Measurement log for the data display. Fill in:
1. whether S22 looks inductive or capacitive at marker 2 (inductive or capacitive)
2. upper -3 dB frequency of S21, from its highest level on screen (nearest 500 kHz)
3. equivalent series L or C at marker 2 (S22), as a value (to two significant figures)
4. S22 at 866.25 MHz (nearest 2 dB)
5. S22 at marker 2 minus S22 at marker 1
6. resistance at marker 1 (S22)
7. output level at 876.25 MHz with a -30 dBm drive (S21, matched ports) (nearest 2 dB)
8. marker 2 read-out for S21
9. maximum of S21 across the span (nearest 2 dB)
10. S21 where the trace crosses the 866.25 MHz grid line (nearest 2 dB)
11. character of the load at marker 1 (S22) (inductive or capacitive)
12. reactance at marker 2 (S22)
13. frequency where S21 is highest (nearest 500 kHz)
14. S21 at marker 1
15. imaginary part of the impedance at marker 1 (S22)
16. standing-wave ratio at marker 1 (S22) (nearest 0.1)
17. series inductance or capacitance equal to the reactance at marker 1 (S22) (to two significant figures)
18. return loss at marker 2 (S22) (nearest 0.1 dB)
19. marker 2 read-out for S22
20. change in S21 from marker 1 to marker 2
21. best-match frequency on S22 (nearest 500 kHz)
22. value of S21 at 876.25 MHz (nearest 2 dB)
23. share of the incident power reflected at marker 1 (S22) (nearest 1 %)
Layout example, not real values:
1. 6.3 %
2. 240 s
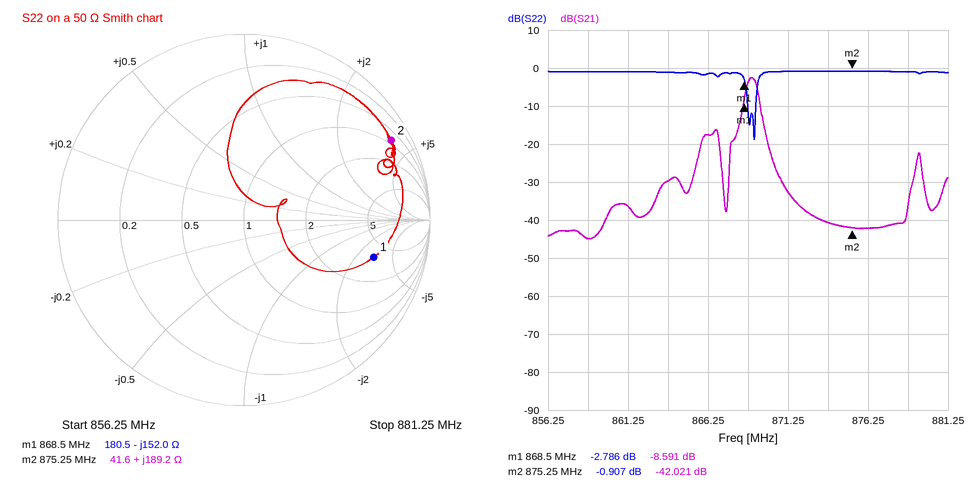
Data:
1. inductive
2. 869.5 MHz
3. 34 nH
4. -2 dB
5. 1.879 dB
6. 180.5 Ω
7. -72 dBm
8. -42.021 dB
9. -2 dB
10. -18 dB
11. capacitive
12. +189.2 Ω
13. 869.0 MHz
14. -8.591 dB
15. -152.0 Ω
16. 6.3
17. 1.2 pF
18. 0.9 dB
19. -0.907 dB
20. -33.430 dB
21. 869.0 MHz
22. -42 dB
23. 53 %
